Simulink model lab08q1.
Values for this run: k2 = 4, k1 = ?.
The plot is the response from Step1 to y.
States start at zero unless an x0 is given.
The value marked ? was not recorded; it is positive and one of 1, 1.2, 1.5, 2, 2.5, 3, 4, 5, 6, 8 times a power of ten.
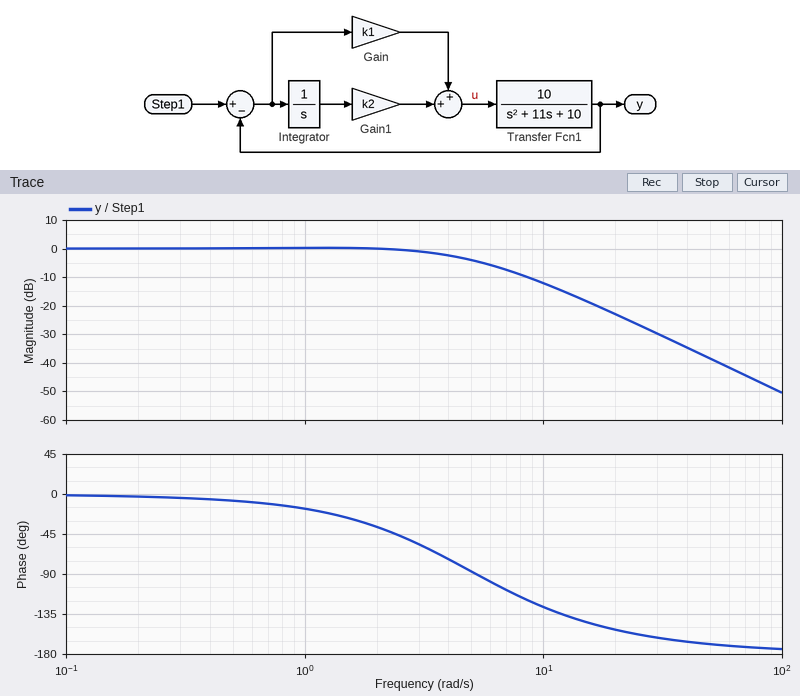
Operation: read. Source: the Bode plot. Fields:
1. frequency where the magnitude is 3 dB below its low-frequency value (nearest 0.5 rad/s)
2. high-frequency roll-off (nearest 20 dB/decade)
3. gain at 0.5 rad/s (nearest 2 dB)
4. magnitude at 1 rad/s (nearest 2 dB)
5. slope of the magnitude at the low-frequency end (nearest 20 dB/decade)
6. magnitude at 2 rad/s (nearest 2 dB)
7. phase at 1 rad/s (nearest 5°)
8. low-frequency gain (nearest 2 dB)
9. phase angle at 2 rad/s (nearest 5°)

4.5 rad/s
-40 dB/decade
0 dB
0 dB
0 dB/decade
0 dB
-15°
0 dB
-35°
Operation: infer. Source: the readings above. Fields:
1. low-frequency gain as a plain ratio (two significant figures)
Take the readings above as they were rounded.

1.0
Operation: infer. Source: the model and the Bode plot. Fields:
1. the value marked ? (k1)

3
